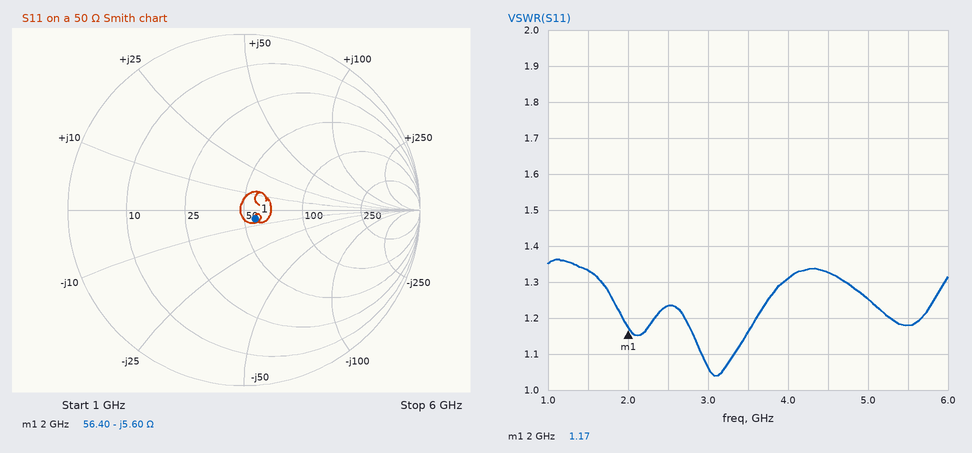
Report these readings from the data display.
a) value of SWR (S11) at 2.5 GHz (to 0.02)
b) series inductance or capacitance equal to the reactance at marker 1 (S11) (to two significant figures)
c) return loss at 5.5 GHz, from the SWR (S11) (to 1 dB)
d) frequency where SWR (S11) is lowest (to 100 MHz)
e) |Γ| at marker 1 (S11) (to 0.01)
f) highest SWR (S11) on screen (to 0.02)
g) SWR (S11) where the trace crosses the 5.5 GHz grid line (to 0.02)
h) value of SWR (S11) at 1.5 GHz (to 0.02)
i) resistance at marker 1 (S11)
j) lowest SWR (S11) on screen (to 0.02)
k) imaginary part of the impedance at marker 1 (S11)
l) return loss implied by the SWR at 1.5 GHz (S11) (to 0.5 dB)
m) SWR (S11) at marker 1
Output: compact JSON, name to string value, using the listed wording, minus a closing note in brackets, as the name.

{"value of SWR (S11) at 2.5 GHz": "1.24", "series inductance or capacitance equal to the reactance at marker 1 (S11)": "14 pF", "return loss at 5.5 GHz, from the SWR (S11)": "22 dB", "frequency where SWR (S11) is lowest": "3.1 GHz", "|Γ| at marker 1 (S11)": "0.08", "highest SWR (S11) on screen": "1.36", "SWR (S11) where the trace crosses the 5.5 GHz grid line": "1.18", "value of SWR (S11) at 1.5 GHz": "1.34", "resistance at marker 1": "56.40 Ω", "lowest SWR (S11) on screen": "1.04", "imaginary part of the impedance at marker 1": "-5.60 Ω", "return loss implied by the SWR at 1.5 GHz (S11)": "17.0 dB", "SWR (S11) at marker 1": "1.17"}
